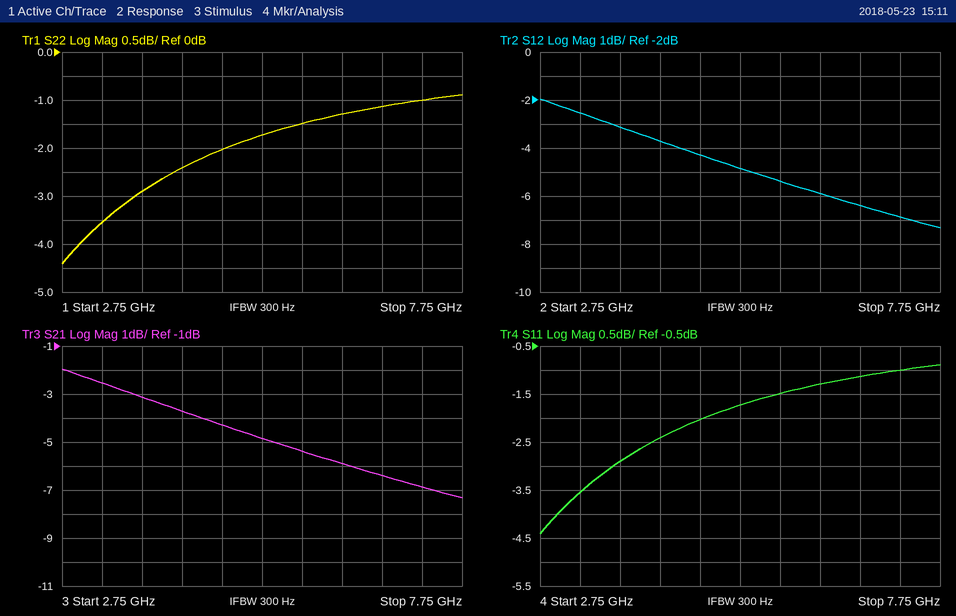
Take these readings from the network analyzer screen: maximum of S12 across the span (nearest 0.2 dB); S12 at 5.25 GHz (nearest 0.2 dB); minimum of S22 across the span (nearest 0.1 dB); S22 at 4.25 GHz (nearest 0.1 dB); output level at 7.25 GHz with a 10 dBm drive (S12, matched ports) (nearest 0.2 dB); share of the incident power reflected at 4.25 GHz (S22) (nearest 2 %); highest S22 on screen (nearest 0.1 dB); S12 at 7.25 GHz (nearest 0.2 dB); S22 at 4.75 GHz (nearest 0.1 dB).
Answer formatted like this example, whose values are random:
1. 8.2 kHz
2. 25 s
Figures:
1. -2.0 dB
2. -4.8 dB
3. -4.4 dB
4. -2.4 dB
5. 3.2 dBm
6. 58 %
7. -0.9 dB
8. -6.8 dB
9. -2.0 dB
